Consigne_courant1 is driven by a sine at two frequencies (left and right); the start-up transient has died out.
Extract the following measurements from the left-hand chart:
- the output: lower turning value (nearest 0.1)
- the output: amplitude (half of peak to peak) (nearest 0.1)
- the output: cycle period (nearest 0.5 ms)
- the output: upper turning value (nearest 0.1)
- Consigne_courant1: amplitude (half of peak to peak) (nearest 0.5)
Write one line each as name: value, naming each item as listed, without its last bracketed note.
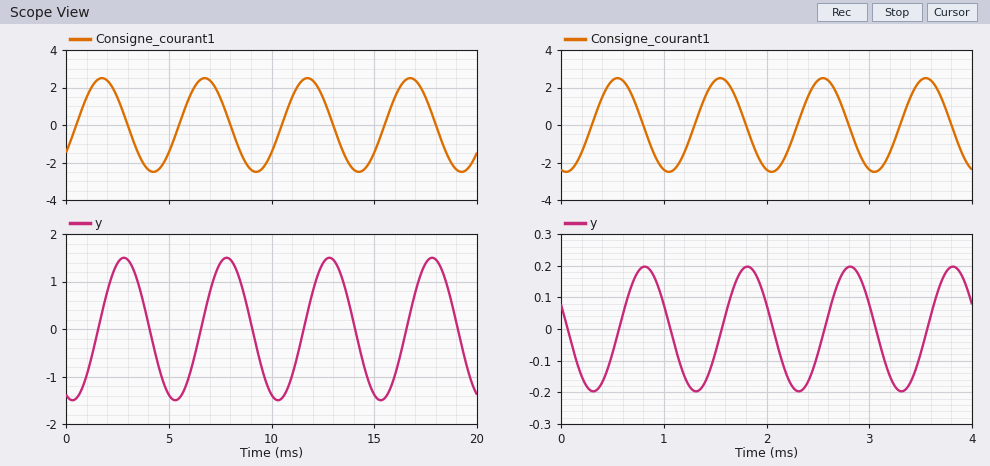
the output: lower turning value: -1.5
the output: amplitude (half of peak to peak): 1.5
the output: cycle period: 5.0 ms
the output: upper turning value: 1.5
Consigne_courant1: amplitude (half of peak to peak): 2.5
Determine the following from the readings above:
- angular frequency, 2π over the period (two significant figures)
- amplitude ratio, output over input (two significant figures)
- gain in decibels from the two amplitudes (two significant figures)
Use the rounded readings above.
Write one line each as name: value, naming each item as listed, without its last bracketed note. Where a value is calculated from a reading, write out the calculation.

angular frequency, 2π over the period: 2π / 5 = 1.3 rad/ms
amplitude ratio, output over input: 1.5 / 2.5 = 0.60
gain in decibels from the two amplitudes: 20 log10(1.5 / 2.5) = -4.4 dB
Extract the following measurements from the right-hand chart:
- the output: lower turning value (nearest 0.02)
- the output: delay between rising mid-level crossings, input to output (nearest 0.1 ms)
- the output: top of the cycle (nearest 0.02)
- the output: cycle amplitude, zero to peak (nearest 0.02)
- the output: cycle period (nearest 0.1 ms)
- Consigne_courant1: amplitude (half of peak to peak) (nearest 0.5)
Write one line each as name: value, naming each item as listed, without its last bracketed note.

the output: lower turning value: -0.20
the output: delay between rising mid-level crossings, input to output: 0.3 ms
the output: top of the cycle: 0.20
the output: cycle amplitude, zero to peak: 0.20
the output: cycle period: 1.0 ms
Consigne_courant1: amplitude (half of peak to peak): 2.5
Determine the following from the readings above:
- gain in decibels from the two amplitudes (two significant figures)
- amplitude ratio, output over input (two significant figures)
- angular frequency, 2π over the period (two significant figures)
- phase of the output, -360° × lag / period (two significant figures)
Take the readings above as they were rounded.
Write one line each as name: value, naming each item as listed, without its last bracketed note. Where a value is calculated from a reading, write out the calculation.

gain in decibels from the two amplitudes: 20 log10(0.2 / 2.5) = -22 dB
amplitude ratio, output over input: 0.2 / 2.5 = 0.080
angular frequency, 2π over the period: 2π / 1 = 6.3 rad/ms
phase of the output, -360° × lag / period: -360 × 0.3 / 1 = -110°
